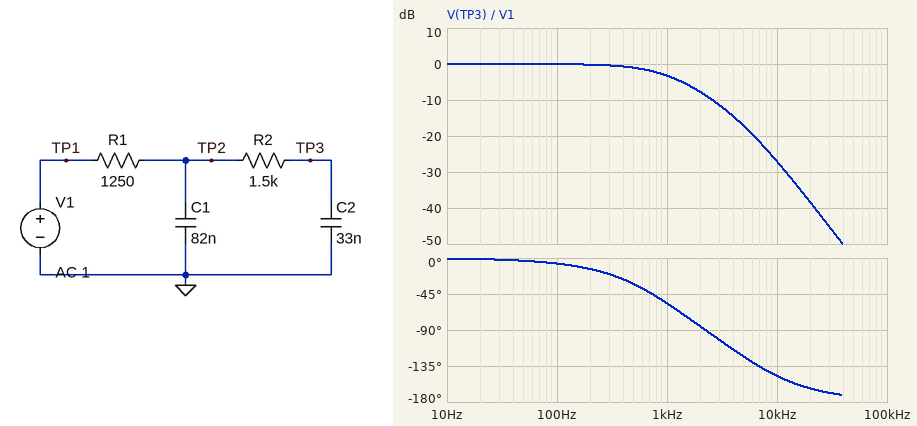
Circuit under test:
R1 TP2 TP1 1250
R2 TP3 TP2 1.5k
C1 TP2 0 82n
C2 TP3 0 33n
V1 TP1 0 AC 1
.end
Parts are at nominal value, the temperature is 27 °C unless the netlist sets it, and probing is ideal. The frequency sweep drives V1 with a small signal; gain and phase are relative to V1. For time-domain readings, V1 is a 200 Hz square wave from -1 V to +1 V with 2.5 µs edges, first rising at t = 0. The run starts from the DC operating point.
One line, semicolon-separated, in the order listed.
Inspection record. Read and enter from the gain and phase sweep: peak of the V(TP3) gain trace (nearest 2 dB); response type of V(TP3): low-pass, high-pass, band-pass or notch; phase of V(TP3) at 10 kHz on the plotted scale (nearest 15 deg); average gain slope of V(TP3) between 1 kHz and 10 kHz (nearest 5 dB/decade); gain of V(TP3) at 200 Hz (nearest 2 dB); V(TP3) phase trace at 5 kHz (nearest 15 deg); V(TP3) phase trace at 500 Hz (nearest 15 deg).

0 dB; low-pass; -150 deg; -25 dB/decade; 0 dB; -120 deg; -30 deg
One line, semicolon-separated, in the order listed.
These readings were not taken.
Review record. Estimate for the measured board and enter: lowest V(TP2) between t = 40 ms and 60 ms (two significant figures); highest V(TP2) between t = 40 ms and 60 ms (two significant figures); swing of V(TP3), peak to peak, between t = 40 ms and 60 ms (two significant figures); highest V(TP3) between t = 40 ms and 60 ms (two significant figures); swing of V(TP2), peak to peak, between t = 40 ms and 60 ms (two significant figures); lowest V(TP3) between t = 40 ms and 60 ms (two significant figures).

-1.0 V; 1.0 V; 2.0 V; 1.0 V; 2.0 V; -1.0 V
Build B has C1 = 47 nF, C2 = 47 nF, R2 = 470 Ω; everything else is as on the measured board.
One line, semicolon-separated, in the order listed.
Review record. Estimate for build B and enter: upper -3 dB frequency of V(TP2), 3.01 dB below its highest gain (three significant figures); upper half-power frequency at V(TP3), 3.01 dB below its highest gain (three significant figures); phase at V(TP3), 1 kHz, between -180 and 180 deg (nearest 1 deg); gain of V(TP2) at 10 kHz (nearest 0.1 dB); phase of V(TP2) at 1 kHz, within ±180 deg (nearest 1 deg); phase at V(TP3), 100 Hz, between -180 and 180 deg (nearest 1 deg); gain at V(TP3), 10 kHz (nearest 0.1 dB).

1.26 kHz; 1.22 kHz; -43 deg; -15.1 dB; -35 deg; -5 deg; -19.7 dB
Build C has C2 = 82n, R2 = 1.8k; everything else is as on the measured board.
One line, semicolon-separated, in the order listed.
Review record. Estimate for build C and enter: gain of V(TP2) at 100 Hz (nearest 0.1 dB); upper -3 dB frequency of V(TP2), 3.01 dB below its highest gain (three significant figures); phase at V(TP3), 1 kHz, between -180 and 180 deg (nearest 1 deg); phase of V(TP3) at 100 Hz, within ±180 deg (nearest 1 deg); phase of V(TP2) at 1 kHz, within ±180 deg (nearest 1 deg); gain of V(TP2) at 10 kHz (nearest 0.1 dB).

-0.1 dB; 681 Hz; -80 deg; -13 deg; -37 deg; -16.6 dB
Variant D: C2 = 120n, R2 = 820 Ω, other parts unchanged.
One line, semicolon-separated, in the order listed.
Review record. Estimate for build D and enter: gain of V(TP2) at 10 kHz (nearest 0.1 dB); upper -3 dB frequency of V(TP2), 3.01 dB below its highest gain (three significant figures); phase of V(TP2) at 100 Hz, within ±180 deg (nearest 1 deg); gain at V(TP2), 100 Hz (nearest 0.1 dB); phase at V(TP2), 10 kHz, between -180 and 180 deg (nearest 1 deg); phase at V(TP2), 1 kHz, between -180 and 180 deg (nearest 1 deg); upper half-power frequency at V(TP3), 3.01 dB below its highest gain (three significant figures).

-17.1 dB; 547 Hz; -9 deg; -0.2 dB; -70 deg; -43 deg; 494 Hz
